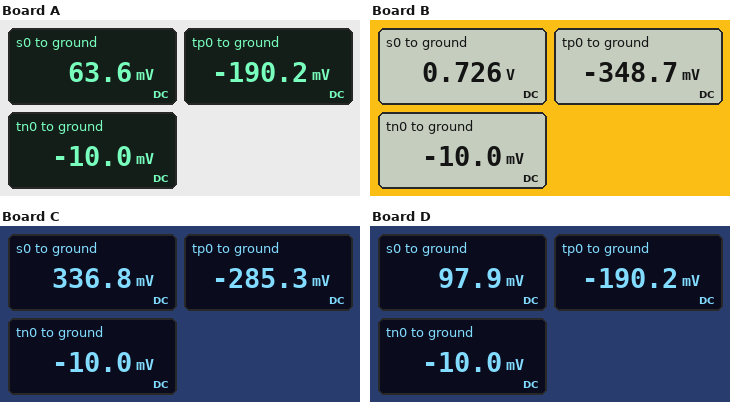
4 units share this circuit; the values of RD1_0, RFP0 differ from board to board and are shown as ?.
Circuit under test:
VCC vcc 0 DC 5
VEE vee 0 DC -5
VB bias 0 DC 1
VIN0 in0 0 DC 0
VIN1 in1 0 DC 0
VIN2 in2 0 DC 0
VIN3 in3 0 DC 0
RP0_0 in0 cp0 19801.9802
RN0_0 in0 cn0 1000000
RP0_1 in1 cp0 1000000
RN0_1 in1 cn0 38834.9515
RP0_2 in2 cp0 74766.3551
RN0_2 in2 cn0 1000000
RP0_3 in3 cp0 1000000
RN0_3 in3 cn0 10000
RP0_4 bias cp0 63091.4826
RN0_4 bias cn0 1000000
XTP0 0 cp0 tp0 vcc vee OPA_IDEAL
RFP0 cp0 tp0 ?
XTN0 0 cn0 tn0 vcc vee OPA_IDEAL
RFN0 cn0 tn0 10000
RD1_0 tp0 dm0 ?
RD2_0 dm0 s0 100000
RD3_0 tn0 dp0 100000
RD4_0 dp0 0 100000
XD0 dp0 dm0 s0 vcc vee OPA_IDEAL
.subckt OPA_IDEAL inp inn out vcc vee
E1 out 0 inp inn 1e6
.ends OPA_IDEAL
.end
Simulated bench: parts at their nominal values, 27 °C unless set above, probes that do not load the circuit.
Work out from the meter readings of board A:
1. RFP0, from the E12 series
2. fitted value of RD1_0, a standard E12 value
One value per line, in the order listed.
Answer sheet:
12 kΩ
270 kΩ
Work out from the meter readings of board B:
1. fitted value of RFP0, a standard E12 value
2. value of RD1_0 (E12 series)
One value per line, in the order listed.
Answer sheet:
22 kΩ
47 kΩ
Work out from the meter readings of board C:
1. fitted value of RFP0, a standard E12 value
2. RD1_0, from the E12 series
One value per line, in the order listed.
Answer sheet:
18 kΩ
82 kΩ
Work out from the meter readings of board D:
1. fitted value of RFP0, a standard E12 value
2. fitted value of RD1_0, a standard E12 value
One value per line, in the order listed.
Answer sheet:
12 kΩ
180 kΩ
